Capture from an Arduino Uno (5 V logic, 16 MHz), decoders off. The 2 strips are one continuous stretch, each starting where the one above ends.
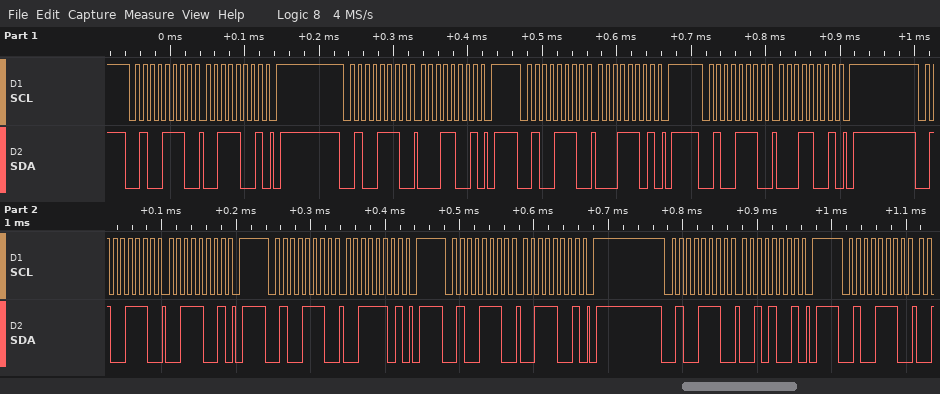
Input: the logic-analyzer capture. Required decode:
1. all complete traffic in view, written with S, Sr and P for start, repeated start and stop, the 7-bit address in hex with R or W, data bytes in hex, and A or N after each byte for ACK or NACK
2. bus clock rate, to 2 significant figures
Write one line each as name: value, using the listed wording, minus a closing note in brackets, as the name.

all complete traffic in view, written with S, Sr and P for start, repeated start and stop, the 7-bit address in hex with R or W, data bytes in hex, and A or N after each byte for ACK or NACK: S 27W A 39 A P S 27W A 19 A P S 27W A 1D A P S 27W A 19 A P S 27W A 39 A P S 27W A 3D A P S 27W A 39 A P S 27W A 29 A P S 27W A
bus clock rate, to 2 significant figures: 100 kHz
